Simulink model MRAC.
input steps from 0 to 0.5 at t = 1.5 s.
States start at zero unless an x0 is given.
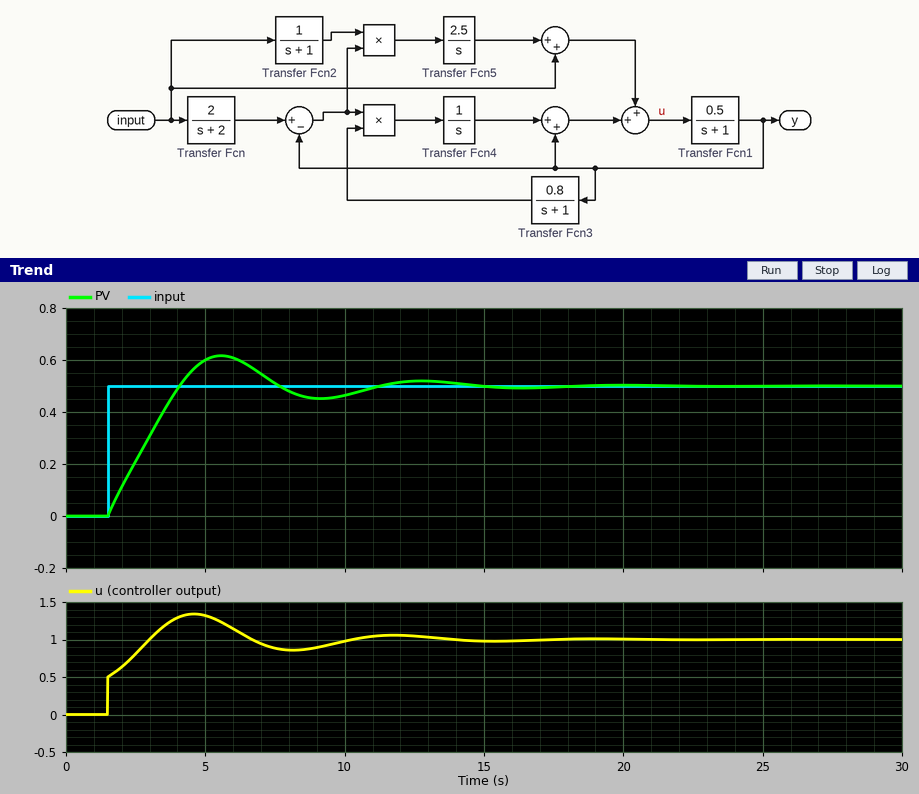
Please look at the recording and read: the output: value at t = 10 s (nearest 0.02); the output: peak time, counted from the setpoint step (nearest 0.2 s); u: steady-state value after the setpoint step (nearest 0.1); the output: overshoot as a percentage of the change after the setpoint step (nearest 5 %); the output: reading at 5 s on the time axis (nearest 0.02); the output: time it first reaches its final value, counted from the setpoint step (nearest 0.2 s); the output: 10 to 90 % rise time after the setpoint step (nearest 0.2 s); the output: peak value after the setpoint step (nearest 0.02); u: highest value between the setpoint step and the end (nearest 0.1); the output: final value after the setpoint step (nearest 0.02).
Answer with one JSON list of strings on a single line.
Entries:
["0.46", "4.0 s", "1.0", "25 %", "0.60", "2.6 s", "2.0 s", "0.62", "1.3", "0.50"]
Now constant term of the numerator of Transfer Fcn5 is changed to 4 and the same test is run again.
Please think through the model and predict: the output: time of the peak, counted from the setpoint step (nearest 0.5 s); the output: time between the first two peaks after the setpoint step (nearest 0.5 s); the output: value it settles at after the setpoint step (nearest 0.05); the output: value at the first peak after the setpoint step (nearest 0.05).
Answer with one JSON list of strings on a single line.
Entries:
["3.5 s", "6.0 s", "0.50", "0.65"]
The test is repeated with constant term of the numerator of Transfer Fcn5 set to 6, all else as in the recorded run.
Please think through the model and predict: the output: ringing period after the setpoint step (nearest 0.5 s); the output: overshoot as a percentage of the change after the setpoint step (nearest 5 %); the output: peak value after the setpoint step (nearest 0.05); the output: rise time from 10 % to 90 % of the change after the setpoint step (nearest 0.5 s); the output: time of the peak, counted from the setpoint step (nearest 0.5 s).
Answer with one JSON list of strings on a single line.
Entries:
["5.0 s", "30 %", "0.65", "1.5 s", "3.0 s"]
